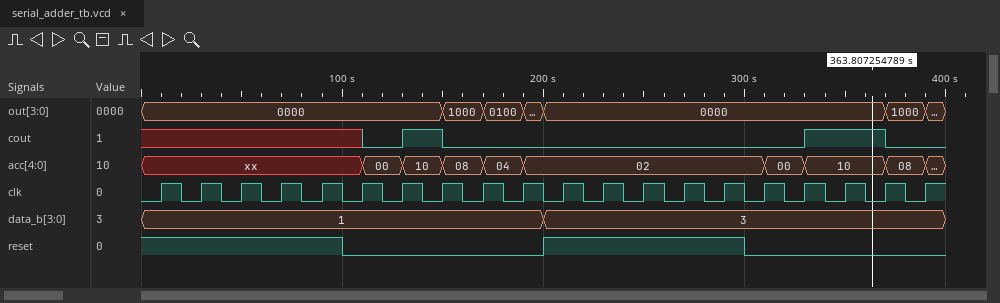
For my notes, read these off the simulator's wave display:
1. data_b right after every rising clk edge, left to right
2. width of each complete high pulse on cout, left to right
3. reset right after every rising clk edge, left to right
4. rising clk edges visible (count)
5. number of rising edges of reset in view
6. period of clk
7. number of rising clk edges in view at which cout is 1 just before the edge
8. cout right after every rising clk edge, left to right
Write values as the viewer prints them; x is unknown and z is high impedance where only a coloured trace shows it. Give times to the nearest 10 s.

1, 1, 1, 1, 1, 1, 1, 1, 1, 1, 3, 3, 3, 3, 3, 3, 3, 3, 3, 3
20 s, 40 s
1 1 1 1 1 0 0 0 0 0 1 1 1 1 1 0 0 0 0 0
20
1
20 s
3
x x x x x 0 1 0 0 0 0 0 0 0 0 0 1 1 0 0
